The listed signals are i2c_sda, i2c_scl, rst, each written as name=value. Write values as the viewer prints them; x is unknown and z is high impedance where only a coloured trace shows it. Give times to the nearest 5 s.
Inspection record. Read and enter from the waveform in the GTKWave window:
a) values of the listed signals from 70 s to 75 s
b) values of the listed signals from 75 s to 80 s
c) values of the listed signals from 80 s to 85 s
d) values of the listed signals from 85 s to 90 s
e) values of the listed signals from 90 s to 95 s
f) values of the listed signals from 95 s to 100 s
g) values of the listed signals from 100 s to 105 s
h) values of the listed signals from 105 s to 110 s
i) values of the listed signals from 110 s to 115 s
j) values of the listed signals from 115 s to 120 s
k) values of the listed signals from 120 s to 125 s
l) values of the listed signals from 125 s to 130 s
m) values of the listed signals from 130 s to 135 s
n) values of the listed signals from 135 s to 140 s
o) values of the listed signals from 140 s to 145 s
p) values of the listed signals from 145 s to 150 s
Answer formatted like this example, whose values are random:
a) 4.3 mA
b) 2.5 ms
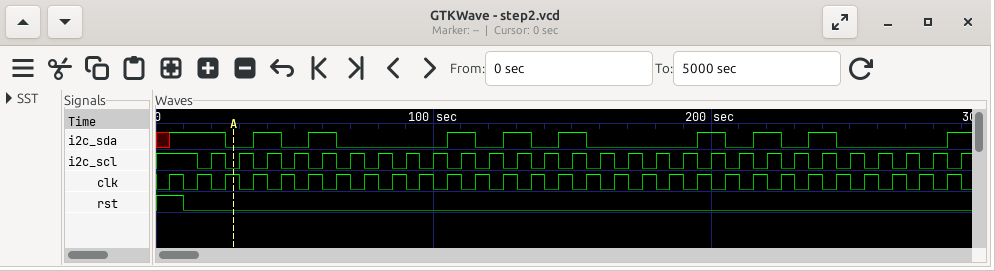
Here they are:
a) i2c_sda=0, i2c_scl=1, rst=0
b) i2c_sda=0, i2c_scl=0, rst=0
c) i2c_sda=0, i2c_scl=1, rst=0
d) i2c_sda=0, i2c_scl=0, rst=0
e) i2c_sda=0, i2c_scl=1, rst=0
f) i2c_sda=0, i2c_scl=0, rst=0
g) i2c_sda=0, i2c_scl=1, rst=0
h) i2c_sda=1, i2c_scl=0, rst=0
i) i2c_sda=1, i2c_scl=1, rst=0
j) i2c_sda=0, i2c_scl=0, rst=0
k) i2c_sda=0, i2c_scl=1, rst=0
l) i2c_sda=1, i2c_scl=0, rst=0
m) i2c_sda=1, i2c_scl=1, rst=0
n) i2c_sda=0, i2c_scl=0, rst=0
o) i2c_sda=0, i2c_scl=1, rst=0
p) i2c_sda=1, i2c_scl=0, rst=0
